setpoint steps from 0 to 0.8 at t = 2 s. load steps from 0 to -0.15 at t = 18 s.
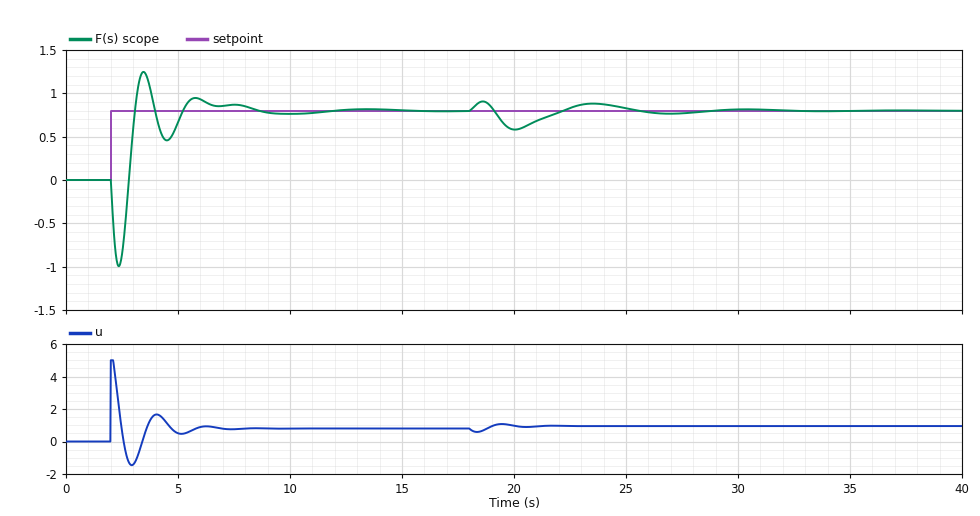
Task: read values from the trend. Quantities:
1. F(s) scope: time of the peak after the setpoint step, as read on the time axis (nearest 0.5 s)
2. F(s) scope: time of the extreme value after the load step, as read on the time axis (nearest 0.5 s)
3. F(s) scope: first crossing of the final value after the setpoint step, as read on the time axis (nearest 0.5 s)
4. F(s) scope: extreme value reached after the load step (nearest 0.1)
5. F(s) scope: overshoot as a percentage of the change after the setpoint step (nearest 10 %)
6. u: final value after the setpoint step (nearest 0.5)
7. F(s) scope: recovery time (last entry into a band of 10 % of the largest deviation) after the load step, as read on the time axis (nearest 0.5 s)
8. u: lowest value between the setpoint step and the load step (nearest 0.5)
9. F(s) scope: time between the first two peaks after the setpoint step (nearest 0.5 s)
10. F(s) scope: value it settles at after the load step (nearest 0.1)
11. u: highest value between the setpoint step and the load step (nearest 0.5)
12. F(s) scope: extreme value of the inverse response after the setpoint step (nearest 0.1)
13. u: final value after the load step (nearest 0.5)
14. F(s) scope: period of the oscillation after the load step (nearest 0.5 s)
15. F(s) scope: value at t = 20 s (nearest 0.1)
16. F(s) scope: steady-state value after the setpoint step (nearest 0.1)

3.5 s
20.0 s
3.0 s
0.6
60 %
1.0
28.0 s
-1.5
2.5 s
0.8
5.0
-1.0
1.0
7.0 s
0.6
0.8
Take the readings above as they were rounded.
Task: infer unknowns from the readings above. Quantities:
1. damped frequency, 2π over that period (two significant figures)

2.5 rad/s
